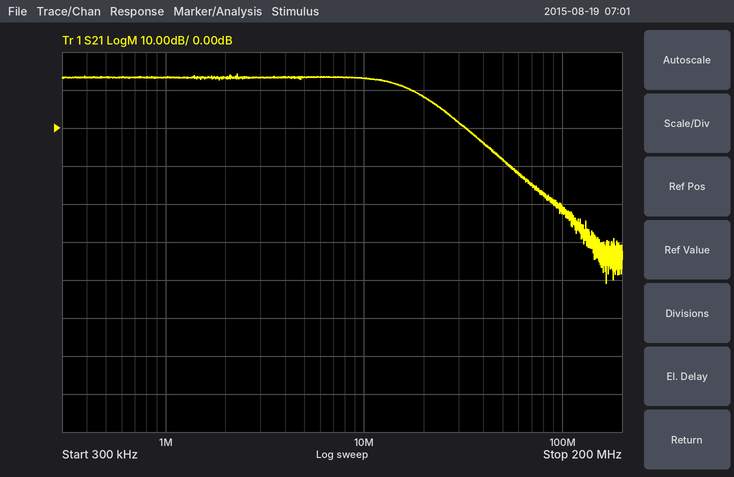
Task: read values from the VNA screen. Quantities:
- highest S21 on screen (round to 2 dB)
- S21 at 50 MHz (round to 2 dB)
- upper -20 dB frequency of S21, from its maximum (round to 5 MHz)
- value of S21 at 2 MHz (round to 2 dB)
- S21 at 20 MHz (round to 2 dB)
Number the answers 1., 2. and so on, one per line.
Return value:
1. 14 dB
2. -8 dB
3. 45 MHz
4. 14 dB
5. 8 dB
